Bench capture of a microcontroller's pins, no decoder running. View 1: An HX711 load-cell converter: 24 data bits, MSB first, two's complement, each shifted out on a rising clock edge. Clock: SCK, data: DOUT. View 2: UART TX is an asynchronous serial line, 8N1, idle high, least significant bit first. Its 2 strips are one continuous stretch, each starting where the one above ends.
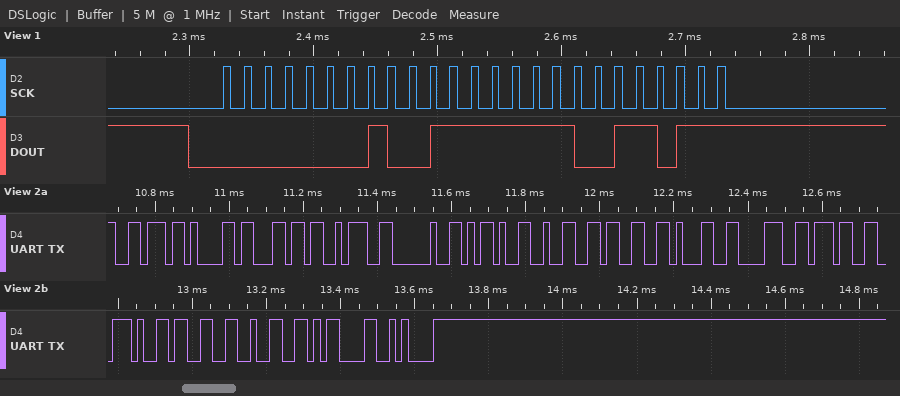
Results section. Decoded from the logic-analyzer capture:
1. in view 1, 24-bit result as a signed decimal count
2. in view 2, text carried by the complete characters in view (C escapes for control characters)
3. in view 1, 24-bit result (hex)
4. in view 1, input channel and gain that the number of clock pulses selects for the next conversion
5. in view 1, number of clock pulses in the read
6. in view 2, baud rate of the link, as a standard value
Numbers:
81819
"val: -23187.32\r\n"
0x013F9B
channel A, gain 128
25
57600 baud
